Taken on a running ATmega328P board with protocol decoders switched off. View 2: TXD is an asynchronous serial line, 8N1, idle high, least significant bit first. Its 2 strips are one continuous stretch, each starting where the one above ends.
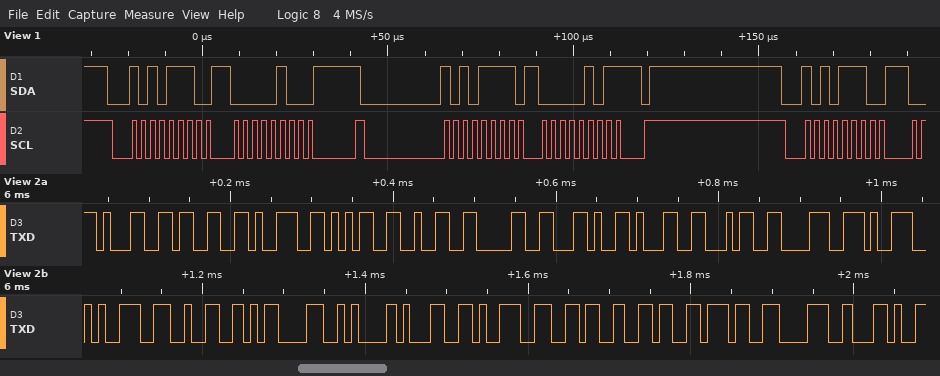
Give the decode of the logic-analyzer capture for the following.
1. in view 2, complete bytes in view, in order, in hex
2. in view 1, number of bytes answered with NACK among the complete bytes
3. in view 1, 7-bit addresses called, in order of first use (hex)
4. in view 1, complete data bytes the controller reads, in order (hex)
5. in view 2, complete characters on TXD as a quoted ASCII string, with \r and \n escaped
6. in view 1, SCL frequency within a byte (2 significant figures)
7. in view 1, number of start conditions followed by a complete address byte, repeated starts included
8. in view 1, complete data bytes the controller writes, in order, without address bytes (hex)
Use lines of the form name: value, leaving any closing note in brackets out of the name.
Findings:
in view 2, complete bytes in view, in order, in hex: 31 33 39 35 32 30 2C 31 34 38 39 39 32 0D 0A 31 39 36 36 37 38 2C
in view 1, number of bytes answered with NACK among the complete bytes: 1
in view 1, 7-bit addresses called, in order of first use: 0x57
in view 1, complete data bytes the controller reads, in order: 05
in view 2, complete characters on TXD as a quoted ASCII string, with \r and \n escaped: "139520,148992\r\n196678,"
in view 1, SCL frequency within a byte: 400 kHz
in view 1, number of start conditions followed by a complete address byte, repeated starts included: 3
in view 1, complete data bytes the controller writes, in order, without address bytes: 04
